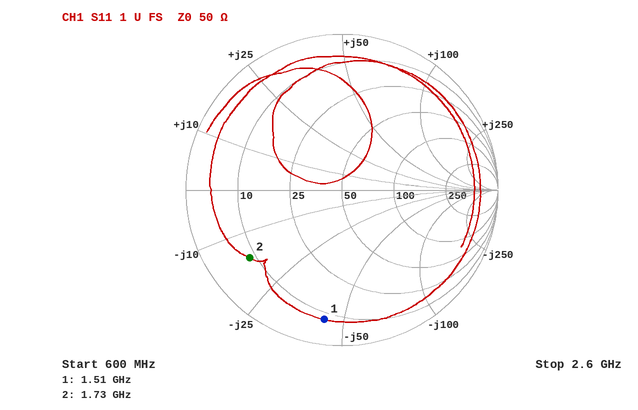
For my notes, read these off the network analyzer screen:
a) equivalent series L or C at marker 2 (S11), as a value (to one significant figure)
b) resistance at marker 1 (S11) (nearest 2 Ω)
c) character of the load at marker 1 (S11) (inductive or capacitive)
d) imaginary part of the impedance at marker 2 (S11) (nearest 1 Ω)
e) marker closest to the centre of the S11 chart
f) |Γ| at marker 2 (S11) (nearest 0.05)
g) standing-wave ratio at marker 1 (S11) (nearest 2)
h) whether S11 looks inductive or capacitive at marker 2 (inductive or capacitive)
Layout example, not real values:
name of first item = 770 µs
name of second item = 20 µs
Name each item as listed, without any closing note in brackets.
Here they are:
equivalent series L or C at marker 2 (S11), as a value = 6 pF
resistance at marker 1 (S11) = 8 Ω
character of the load at marker 1 (S11) = capacitive
imaginary part of the impedance at marker 2 (S11) = -16 Ω
marker closest to the centre of the S11 chart = marker 2
|Γ| at marker 2 (S11) = 0.75
standing-wave ratio at marker 1 (S11) = 12
whether S11 looks inductive or capacitive at marker 2 = capacitive
